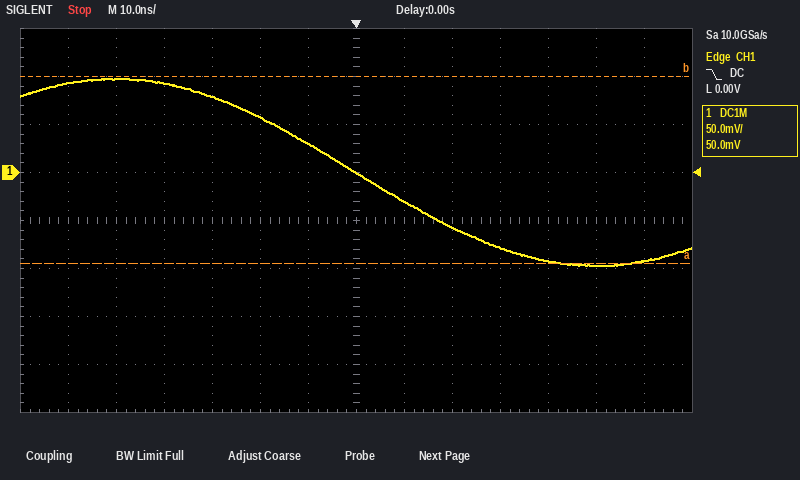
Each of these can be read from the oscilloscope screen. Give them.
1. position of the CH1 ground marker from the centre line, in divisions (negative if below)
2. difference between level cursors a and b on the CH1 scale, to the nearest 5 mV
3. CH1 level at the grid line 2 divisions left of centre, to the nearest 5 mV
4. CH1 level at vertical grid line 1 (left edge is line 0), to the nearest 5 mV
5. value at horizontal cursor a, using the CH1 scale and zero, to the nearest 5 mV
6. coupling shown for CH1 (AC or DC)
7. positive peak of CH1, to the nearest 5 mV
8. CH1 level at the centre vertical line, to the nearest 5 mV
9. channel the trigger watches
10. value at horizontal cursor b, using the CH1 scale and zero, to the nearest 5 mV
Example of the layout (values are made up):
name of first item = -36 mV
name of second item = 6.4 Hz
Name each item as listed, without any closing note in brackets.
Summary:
position of the CH1 ground marker from the centre line, in divisions = +1.0 div
difference between level cursors a and b on the CH1 scale, to the nearest 5 mV = 195 mV
CH1 level at the grid line 2 divisions left of centre, to the nearest 5 mV = 60 mV
CH1 level at vertical grid line 1 (left edge is line 0), to the nearest 5 mV = 95 mV
value at horizontal cursor a, using the CH1 scale and zero, to the nearest 5 mV = -95 mV
coupling shown for CH1 = DC
positive peak of CH1, to the nearest 5 mV = 100 mV
CH1 level at the centre vertical line, to the nearest 5 mV = 0 mV
channel the trigger watches = CH1
value at horizontal cursor b, using the CH1 scale and zero, to the nearest 5 mV = 100 mV
